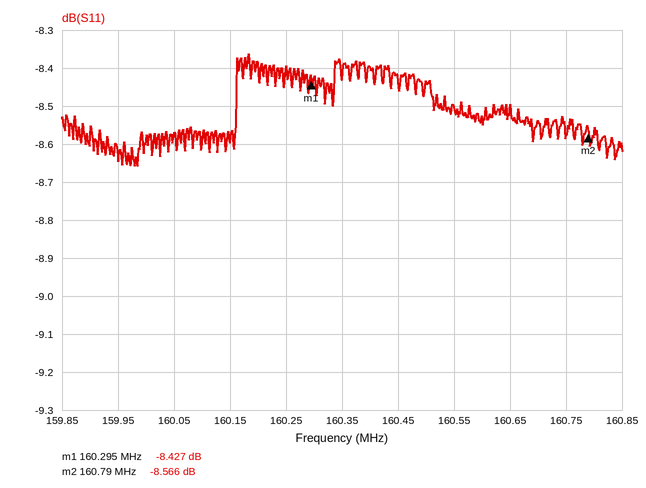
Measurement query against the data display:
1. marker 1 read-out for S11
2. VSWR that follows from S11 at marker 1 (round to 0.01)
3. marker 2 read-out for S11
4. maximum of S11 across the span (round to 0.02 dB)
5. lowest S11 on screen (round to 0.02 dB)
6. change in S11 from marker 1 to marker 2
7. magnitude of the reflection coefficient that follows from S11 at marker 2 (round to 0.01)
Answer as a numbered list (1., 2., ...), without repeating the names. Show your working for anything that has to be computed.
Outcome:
1. -8.427 dB
2. (1 + 0.3790)/(1 − 0.3790) ≈ 2.22
3. -8.566 dB
4. -8.36 dB
5. -8.66 dB
6. -8.566 − (-8.427) = -0.139 dB
7. 10^(-8.566/20) ≈ 0.37
